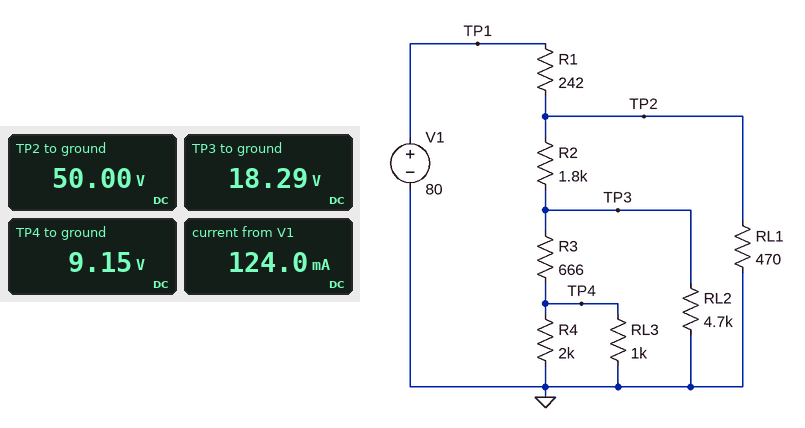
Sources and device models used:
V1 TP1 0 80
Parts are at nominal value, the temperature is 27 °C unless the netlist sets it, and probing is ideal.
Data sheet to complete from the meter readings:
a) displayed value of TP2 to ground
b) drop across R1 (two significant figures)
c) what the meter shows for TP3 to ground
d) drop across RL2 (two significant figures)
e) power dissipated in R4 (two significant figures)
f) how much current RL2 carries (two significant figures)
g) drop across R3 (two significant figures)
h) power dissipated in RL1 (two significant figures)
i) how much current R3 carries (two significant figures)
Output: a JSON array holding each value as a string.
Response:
["50.00 V", "30 V", "18.29 V", "18 V", "42 mW", "3.9 mA", "9.1 V", "5.3 W", "14 mA"]
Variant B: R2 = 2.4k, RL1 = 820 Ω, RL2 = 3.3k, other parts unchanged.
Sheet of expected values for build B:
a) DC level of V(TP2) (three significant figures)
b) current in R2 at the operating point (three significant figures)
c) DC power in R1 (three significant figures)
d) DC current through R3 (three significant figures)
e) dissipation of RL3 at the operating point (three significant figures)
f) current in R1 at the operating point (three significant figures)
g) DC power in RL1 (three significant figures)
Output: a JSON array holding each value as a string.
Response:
["58.5 V", "17.5 mA", "1.91 W", "12.4 mA", "68.8 mW", "88.8 mA", "4.17 W"]
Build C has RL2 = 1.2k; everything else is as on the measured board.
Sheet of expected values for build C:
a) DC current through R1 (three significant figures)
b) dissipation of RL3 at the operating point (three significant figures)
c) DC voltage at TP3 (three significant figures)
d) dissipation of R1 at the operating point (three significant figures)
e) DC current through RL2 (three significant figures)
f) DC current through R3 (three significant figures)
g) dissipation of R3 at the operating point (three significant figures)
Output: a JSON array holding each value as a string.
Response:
["126 mA", "41.4 mW", "12.9 V", "3.83 W", "10.7 mA", "9.66 mA", "62.1 mW"]
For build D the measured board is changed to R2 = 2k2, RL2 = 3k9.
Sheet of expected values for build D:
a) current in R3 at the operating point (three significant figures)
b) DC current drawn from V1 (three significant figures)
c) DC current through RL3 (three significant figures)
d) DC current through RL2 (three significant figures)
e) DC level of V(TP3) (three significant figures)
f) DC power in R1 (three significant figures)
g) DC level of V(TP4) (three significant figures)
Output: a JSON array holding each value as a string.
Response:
["11.7 mA", "123 mA", "7.83 mA", "4.01 mA", "15.6 V", "3.65 W", "7.83 V"]
